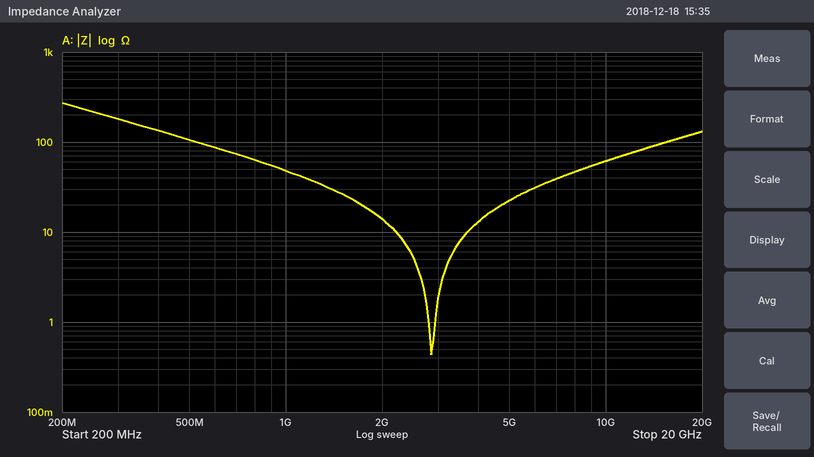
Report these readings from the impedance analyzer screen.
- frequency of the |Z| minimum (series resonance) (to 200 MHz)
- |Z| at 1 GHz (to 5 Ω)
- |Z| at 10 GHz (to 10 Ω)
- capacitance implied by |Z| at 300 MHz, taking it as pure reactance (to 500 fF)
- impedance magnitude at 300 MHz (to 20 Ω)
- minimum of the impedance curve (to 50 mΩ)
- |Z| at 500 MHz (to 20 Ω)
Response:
2.8 GHz
50 Ω
60 Ω
3.0 pF
180 Ω
450 mΩ
100 Ω
